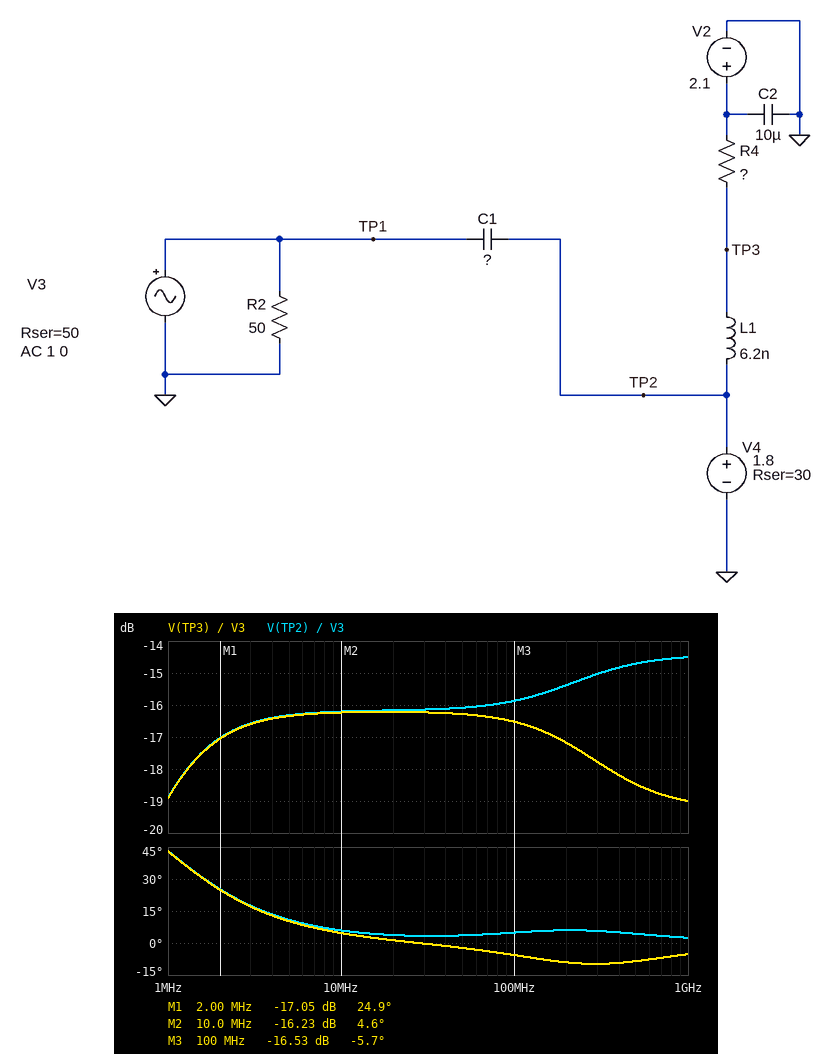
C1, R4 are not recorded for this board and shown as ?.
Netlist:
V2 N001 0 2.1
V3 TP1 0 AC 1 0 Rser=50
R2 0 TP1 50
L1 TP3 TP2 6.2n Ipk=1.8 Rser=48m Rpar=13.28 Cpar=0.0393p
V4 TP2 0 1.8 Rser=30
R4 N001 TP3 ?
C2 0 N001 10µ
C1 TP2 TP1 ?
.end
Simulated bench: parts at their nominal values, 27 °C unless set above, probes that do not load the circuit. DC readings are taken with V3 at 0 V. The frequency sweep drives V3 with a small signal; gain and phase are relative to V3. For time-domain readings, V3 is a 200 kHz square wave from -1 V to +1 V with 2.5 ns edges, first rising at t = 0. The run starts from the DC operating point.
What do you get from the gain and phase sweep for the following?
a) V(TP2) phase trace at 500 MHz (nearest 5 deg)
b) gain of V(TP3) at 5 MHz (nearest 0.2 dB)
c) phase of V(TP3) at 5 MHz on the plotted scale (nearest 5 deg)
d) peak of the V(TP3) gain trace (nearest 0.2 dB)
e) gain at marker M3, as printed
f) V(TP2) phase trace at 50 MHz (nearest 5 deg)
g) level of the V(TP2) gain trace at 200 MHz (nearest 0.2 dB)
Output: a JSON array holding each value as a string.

["5 deg", "-16.4 dB", "10 deg", "-16.2 dB", "-16.53 dB", "5 deg", "-15.4 dB"]
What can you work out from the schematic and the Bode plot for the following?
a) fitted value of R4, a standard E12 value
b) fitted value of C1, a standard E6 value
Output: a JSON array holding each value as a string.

["18 Ω", "4.7 nF"]
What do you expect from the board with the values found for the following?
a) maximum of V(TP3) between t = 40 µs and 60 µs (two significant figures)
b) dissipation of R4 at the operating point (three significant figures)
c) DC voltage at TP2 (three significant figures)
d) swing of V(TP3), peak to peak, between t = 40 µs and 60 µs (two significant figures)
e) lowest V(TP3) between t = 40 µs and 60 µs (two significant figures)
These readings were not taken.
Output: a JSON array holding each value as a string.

["2.3 V", "702 µW", "1.99 V", "610 mV", "1.7 V"]
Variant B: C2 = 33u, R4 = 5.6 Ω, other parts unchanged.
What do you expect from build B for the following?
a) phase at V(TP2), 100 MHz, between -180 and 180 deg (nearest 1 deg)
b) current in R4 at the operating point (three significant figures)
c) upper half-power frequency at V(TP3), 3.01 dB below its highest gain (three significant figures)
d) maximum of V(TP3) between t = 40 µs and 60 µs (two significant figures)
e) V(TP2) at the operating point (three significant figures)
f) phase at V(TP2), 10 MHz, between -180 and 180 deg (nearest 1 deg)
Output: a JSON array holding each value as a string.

["19 deg", "8.42 mA", "378 MHz", "2.2 V", "2.05 V", "9 deg"]
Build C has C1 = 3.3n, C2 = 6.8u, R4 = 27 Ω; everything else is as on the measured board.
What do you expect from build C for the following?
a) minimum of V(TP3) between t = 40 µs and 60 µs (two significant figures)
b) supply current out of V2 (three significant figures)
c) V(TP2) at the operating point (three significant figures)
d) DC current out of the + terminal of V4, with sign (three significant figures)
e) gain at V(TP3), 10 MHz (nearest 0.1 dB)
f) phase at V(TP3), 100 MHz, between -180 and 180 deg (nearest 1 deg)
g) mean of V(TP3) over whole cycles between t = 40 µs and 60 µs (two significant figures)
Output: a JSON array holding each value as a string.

["1.6 V", "5.26 mA", "1.96 V", "-5.26 mA", "-14.9 dB", "-4 deg", "2.0 V"]
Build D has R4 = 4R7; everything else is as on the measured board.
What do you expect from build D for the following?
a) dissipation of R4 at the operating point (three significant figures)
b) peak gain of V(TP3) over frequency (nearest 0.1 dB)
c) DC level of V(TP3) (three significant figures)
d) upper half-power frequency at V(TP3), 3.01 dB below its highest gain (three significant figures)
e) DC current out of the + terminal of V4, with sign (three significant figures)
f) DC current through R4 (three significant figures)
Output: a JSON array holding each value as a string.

["350 µW", "-23.2 dB", "2.06 V", "355 MHz", "-8.63 mA", "8.63 mA"]
